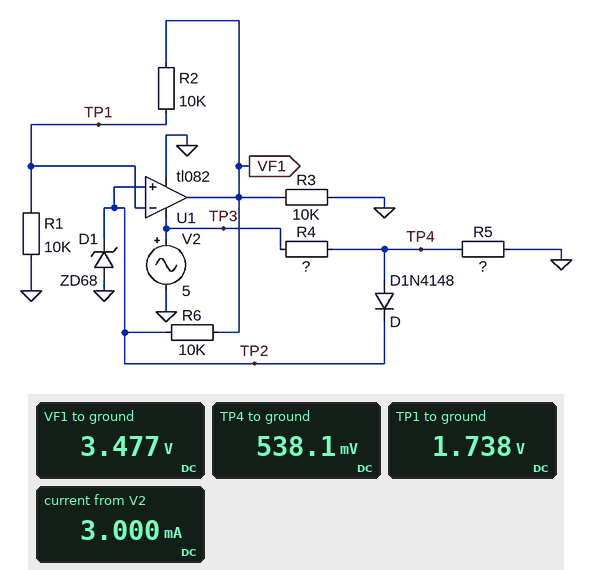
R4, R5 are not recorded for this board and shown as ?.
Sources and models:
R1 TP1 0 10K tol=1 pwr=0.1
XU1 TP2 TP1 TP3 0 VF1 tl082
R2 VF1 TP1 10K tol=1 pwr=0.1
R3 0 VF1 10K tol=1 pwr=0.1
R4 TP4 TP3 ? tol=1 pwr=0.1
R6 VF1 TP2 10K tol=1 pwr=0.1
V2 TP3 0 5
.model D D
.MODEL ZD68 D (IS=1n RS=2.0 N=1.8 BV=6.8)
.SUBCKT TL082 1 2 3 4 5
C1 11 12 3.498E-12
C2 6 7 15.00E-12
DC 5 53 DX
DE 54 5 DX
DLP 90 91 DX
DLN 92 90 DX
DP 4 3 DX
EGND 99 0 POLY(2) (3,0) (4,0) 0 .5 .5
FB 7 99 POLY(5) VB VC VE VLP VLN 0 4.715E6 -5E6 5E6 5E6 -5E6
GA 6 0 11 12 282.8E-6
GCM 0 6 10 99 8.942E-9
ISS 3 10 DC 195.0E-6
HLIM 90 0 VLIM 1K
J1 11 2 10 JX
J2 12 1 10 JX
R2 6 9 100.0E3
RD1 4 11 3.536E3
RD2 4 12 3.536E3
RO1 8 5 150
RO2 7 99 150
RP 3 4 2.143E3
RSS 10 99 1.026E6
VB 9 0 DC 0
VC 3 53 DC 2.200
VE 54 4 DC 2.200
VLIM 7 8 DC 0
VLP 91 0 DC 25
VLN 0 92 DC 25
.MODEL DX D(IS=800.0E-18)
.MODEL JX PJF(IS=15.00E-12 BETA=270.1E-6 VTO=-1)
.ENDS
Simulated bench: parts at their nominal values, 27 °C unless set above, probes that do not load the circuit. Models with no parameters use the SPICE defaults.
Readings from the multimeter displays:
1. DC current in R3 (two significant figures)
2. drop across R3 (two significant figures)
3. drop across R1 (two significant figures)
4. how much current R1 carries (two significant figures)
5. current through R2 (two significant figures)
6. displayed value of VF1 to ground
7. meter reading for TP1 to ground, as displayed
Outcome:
350 µA
3.5 V
1.7 V
170 µA
170 µA
3.477 V
1.738 V
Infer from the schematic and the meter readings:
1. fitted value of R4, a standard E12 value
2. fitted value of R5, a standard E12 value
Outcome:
6.8 kΩ
820 Ω
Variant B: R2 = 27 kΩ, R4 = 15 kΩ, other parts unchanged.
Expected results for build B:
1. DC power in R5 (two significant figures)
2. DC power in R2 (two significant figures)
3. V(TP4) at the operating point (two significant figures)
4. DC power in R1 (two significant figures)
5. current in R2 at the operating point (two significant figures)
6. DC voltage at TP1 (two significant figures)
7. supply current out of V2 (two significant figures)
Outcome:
82 µW
240 µW
260 mV
88 µW
94 µA
940 mV
2.7 mA
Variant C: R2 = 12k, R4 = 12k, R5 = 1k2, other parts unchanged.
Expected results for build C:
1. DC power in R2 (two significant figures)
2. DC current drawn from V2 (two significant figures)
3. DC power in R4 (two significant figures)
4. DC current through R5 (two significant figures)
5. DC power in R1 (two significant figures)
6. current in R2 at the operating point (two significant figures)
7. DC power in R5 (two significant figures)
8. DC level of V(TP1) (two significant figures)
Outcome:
300 µW
2.7 mA
1.7 mW
380 µA
250 µW
160 µA
170 µW
1.6 V
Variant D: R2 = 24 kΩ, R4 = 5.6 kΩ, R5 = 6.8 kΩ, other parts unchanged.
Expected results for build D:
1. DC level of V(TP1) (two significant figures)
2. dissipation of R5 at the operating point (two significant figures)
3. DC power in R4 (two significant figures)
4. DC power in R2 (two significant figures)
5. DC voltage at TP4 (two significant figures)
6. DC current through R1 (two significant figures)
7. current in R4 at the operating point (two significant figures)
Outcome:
1.0 V
1.1 mW
910 µW
250 µW
2.7 V
100 µA
400 µA
